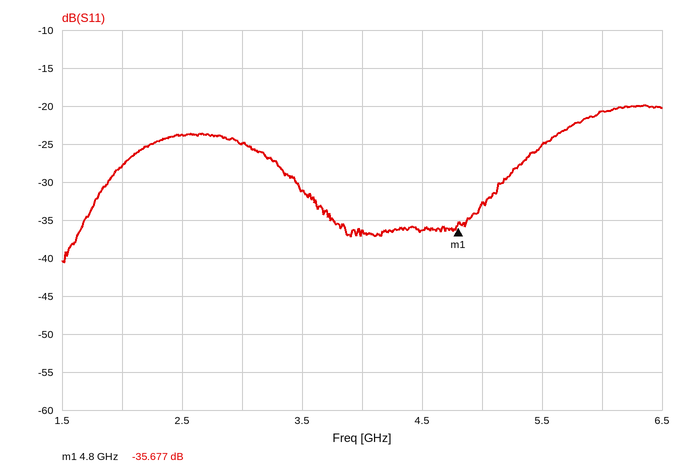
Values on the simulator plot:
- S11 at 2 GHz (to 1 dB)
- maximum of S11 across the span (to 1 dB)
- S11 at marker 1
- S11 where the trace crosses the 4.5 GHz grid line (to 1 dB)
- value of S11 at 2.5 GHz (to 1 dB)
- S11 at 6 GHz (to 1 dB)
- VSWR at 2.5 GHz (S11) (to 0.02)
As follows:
-28 dB
-20 dB
-35.677 dB
-36 dB
-24 dB
-21 dB
1.14
